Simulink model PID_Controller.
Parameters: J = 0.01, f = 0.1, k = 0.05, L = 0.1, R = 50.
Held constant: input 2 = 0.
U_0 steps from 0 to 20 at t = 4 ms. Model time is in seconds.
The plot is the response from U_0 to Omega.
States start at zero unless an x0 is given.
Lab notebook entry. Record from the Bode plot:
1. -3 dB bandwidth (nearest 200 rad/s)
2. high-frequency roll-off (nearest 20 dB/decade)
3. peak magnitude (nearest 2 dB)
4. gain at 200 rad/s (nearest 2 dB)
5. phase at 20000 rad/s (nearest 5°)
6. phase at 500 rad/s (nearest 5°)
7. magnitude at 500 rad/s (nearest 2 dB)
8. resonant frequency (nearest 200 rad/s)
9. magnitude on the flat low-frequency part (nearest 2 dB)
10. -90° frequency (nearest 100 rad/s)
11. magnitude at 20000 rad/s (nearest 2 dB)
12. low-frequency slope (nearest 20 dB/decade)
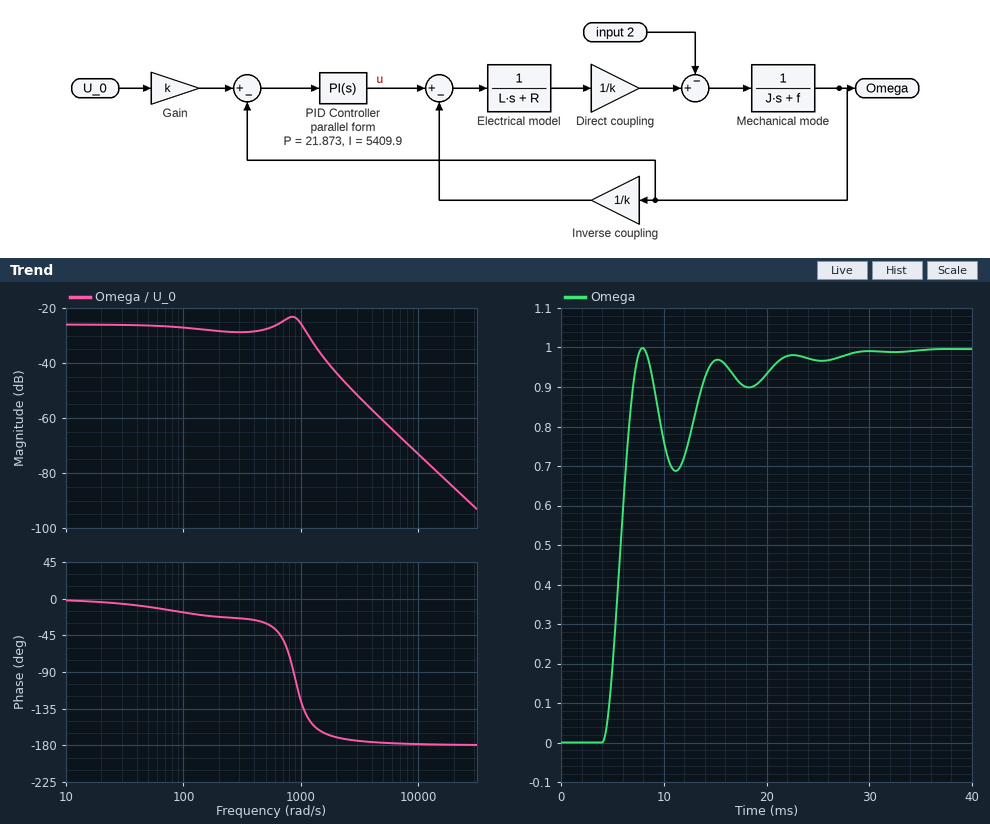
1200 rad/s
-40 dB/decade
-24 dB
-28 dB
-180°
-30°
-28 dB
800 rad/s
-26 dB
900 rad/s
-86 dB
0 dB/decade
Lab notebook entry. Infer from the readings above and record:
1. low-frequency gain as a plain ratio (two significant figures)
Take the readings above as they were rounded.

0.050
